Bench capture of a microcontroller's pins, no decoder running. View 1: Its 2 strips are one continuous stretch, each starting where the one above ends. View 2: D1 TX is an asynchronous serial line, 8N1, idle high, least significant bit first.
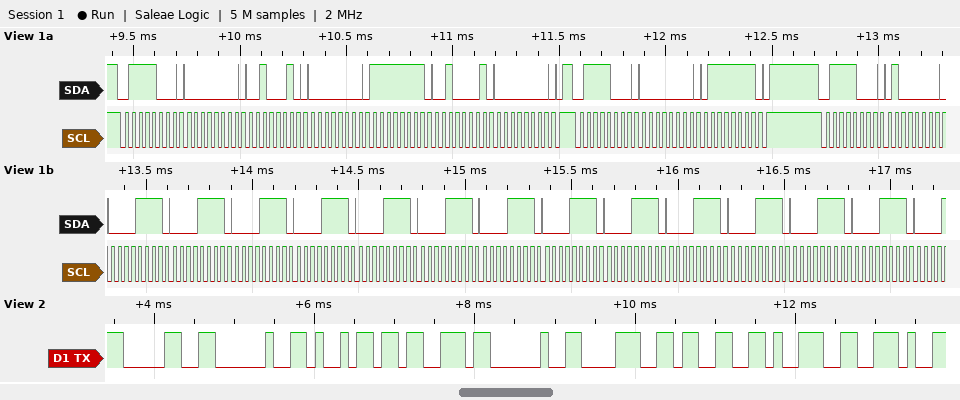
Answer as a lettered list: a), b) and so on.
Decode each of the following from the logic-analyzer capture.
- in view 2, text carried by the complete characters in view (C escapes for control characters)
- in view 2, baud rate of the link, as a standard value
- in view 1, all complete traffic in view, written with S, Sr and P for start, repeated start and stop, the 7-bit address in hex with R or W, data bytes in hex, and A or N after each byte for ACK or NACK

a) "0 is 839."
b) 9600 baud
c) S 3CW A 00 A 22 A 00 A FF A 21 A 00 A P S 3CW A 00 A 7F A P S 3CW A 40 A 0F A 0F A 0F A 0F A 0F A 0F A 0F A 0F A 0F A 0F A 0F A 0F A 0F A
